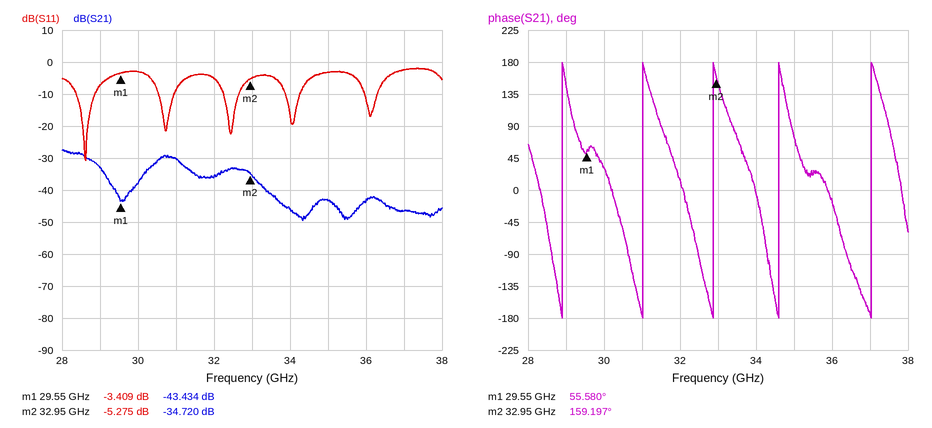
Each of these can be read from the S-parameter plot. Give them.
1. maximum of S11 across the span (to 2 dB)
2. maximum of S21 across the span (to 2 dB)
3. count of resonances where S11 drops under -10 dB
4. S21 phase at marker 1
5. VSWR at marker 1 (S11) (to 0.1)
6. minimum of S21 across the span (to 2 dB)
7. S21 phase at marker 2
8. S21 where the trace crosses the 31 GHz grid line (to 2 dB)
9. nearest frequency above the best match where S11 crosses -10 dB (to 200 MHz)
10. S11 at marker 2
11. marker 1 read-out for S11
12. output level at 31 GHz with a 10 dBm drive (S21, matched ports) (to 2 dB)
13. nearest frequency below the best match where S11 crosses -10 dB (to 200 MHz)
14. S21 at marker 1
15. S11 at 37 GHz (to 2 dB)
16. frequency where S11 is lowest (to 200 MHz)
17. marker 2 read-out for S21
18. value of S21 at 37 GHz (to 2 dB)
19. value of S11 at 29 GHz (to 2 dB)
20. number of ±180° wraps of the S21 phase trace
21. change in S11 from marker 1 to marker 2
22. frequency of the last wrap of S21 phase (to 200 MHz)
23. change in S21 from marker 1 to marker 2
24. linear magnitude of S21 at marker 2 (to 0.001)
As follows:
-2 dB
-28 dB
5
55.580°
5.2
-50 dB
159.197°
-30 dB
28.8 GHz
-5.275 dB
-3.409 dB
-20 dBm
28.4 GHz
-43.434 dB
-2 dB
28.6 GHz
-34.720 dB
-46 dB
-8 dB
5
-1.866 dB
37.0 GHz
8.714 dB
0.018
